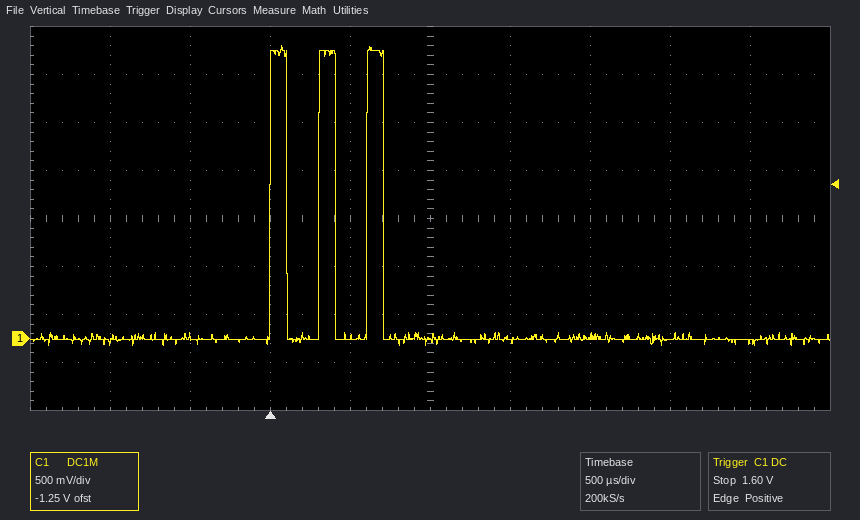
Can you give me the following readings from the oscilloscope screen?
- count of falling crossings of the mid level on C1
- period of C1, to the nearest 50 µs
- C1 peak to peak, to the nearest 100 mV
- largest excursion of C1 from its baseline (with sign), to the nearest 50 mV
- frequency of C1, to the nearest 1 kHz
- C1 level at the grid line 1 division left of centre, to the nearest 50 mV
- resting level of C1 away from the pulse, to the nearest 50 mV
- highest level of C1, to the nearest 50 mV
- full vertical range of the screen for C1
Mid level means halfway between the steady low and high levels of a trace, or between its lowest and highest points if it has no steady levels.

3
300 µs
3.10 V
+3.05 V
3 kHz
0 mV
0 mV
3.05 V
4 V
